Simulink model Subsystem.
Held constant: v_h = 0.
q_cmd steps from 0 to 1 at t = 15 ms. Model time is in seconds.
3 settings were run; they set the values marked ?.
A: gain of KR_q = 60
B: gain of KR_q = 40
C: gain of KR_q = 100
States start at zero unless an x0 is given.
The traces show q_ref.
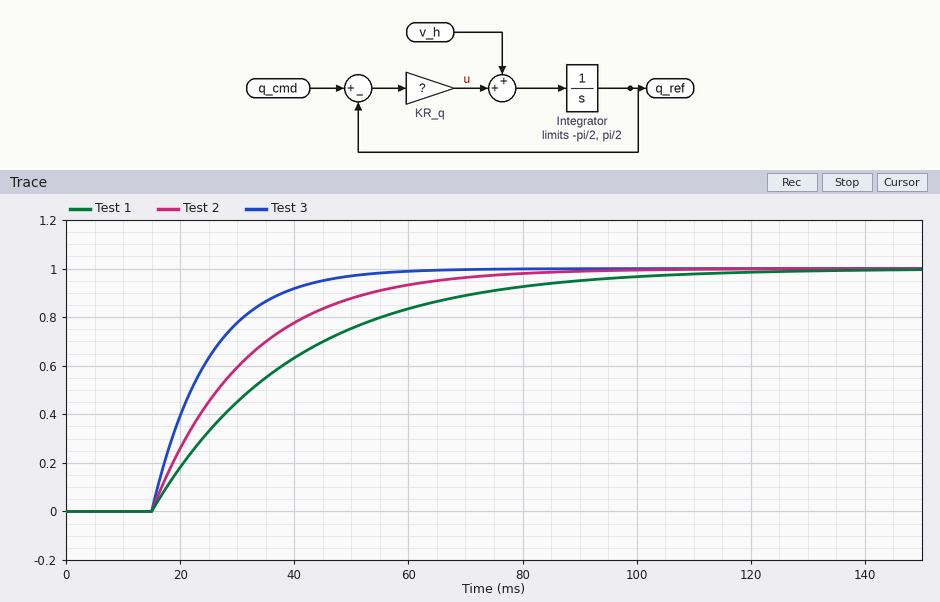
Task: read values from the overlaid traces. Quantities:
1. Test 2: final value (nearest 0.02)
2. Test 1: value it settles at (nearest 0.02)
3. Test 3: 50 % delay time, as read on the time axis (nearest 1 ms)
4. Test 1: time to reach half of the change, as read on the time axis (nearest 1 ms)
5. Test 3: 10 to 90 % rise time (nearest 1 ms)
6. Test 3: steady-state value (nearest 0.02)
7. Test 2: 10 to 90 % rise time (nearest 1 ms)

1.00
1.00
22 ms
32 ms
22 ms
1.00
37 ms
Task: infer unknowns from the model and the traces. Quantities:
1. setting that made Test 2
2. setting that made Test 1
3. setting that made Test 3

A
B
C
